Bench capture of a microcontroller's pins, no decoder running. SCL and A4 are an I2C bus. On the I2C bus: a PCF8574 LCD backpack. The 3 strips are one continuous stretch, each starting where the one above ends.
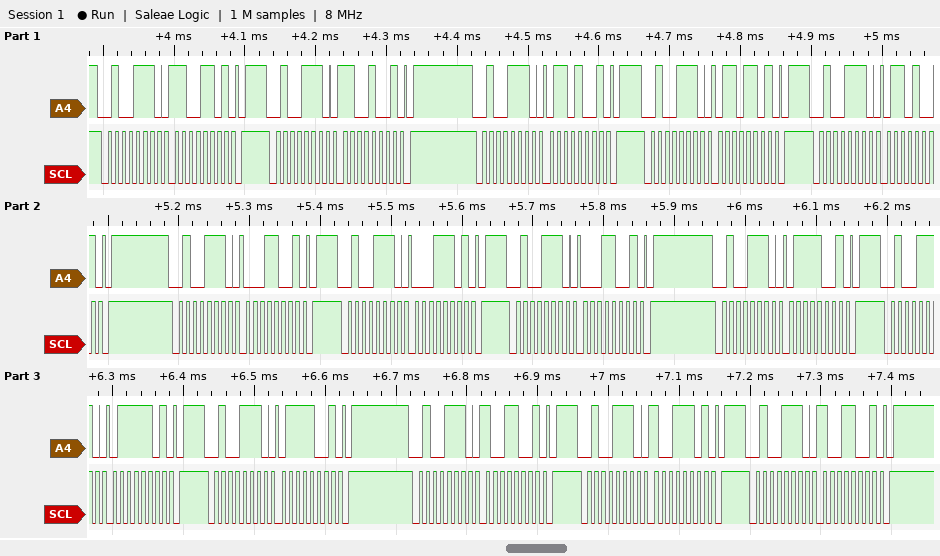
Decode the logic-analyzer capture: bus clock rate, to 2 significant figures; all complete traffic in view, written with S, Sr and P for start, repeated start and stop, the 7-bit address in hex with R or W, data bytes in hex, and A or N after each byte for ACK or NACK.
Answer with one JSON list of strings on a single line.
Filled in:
["100 kHz", "S 27W A CD A P S 27W A C9 A P S 27W A 69 A P S 27W A 6D A P S 27W A 69 A P S 27W A 19 A P S 27W A 1D A P S 27W A 19 A P S 27W A 79 A P S 27W A 7D A P S 27W A 79 A P S 27W A 99 A P S 27W A 9D A P S 27W A 99 A P"]
